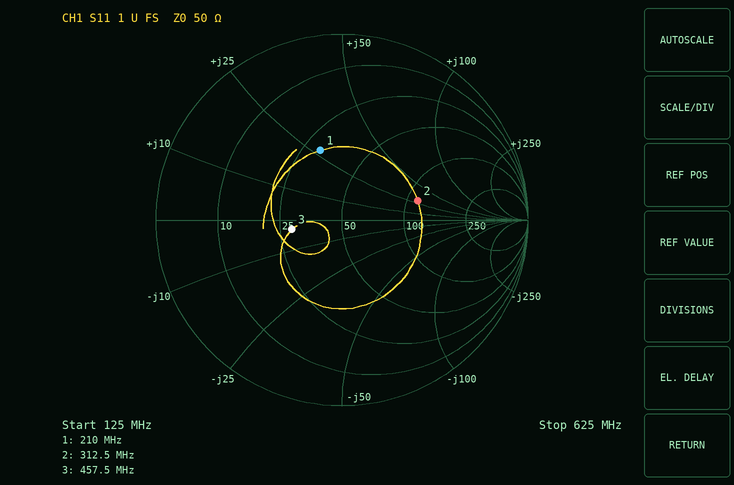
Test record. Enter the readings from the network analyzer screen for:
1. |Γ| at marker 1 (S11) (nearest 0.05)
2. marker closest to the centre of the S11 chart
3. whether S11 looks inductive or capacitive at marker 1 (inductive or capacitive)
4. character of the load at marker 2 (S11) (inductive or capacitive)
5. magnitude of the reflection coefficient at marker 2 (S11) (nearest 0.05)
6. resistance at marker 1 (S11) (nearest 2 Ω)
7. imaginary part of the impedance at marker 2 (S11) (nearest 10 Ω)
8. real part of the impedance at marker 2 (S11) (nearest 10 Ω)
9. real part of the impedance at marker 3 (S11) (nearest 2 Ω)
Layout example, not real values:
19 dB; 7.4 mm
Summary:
0.40; marker 3; inductive; inductive; 0.40; 30 Ω; +30 Ω; 110 Ω; 28 Ω
